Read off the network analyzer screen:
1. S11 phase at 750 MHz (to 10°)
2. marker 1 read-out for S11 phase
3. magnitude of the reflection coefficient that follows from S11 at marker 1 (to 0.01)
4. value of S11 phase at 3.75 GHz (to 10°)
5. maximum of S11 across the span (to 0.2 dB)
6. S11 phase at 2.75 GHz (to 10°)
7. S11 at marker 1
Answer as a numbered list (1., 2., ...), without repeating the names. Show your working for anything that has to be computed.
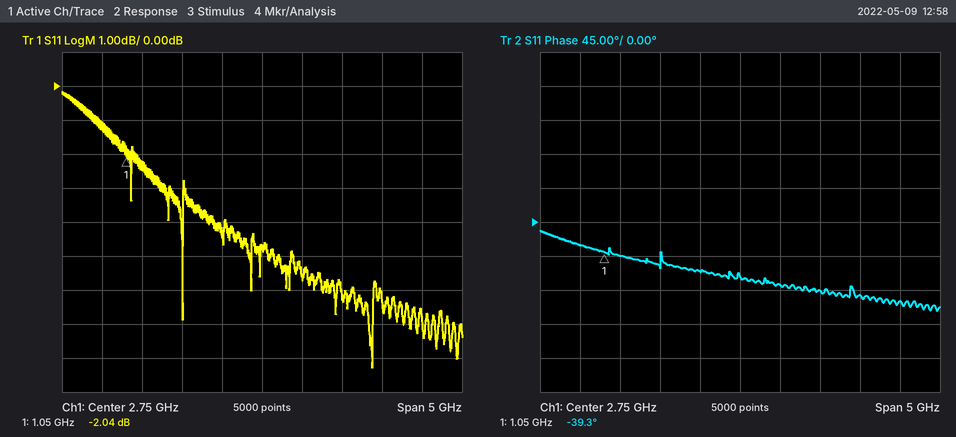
1. -30°
2. -39.3°
3. 10^(-2.04/20) ≈ 0.79
4. -90°
5. -0.2 dB
6. -70°
7. -2.04 dB
